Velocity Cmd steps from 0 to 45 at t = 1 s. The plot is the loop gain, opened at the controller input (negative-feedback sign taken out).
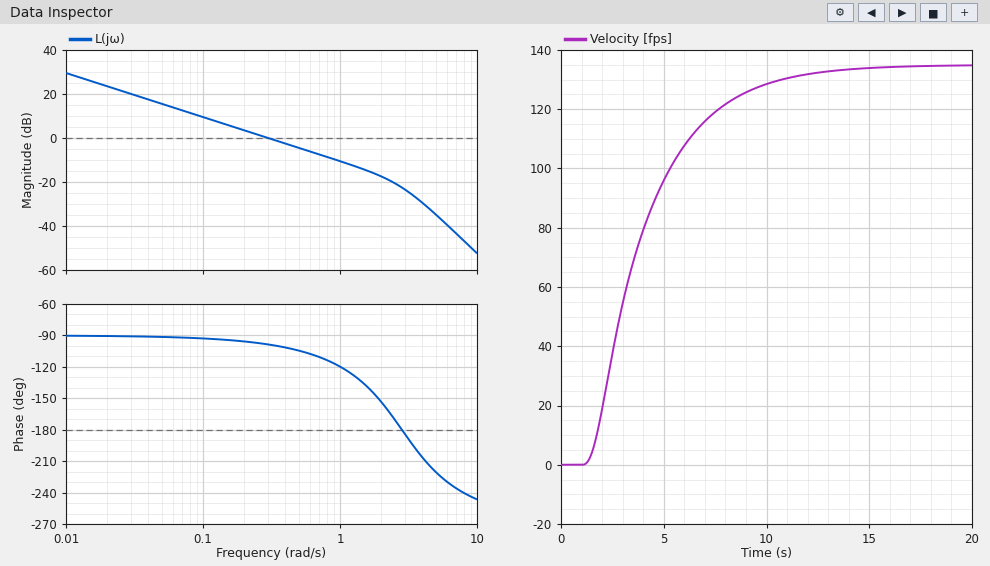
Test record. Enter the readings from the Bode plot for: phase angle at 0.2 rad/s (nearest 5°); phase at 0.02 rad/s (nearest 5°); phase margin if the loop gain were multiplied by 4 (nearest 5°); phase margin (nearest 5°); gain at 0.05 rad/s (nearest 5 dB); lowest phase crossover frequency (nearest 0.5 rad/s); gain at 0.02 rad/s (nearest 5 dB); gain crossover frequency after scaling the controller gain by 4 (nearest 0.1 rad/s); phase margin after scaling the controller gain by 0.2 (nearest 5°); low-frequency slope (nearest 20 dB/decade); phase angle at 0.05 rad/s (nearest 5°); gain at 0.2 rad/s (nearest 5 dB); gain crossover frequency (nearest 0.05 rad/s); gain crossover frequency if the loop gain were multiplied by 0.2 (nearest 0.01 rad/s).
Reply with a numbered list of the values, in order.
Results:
1. -95°
2. -90°
3. 55°
4. 80°
5. 15 dB
6. 3.0 rad/s
7. 25 dB
8. 1.2 rad/s
9. 90°
10. -20 dB/decade
11. -90°
12. 5 dB
13. 0.30 rad/s
14. 0.06 rad/s
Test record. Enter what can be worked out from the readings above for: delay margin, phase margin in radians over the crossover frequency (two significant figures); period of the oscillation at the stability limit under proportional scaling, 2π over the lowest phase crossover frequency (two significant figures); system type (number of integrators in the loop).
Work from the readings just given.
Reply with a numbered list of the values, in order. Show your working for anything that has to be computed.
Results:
1. 80 × π / 180 / 0.3 = 4.7 s
2. 2π / 3 = 2.1 s
3. 1
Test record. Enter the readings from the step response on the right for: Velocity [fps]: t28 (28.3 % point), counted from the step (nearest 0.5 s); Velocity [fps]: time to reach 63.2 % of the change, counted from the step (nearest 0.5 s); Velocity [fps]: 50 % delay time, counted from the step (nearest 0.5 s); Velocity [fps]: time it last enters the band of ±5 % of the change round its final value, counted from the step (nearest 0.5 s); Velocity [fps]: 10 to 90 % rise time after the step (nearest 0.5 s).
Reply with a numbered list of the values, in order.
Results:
1. 1.5 s
2. 3.5 s
3. 2.5 s
4. 9.0 s
5. 6.0 s
